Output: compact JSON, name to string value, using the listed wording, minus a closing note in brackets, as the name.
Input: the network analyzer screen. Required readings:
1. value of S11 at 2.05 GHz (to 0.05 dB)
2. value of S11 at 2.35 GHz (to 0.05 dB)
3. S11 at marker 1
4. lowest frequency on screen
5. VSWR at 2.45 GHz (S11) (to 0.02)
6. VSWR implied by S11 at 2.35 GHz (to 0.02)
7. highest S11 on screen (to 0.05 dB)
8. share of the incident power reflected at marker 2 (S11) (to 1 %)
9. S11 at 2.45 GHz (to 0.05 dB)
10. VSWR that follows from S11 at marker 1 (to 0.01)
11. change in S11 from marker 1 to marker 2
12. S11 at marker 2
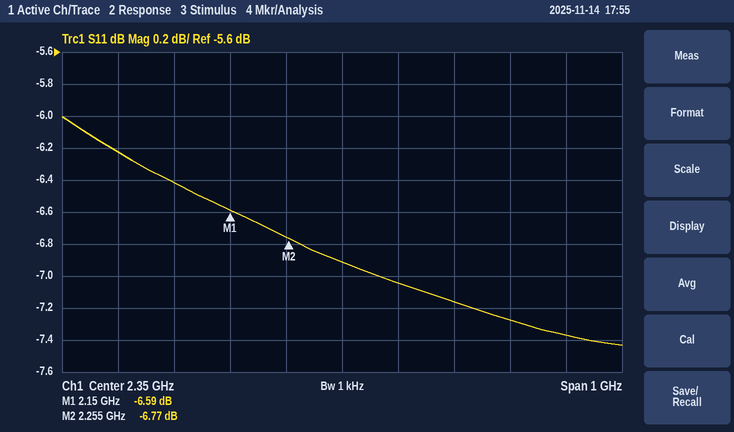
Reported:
{"value of S11 at 2.05 GHz": "-6.40 dB", "value of S11 at 2.35 GHz": "-6.90 dB", "S11 at marker 1": "-6.59 dB", "lowest frequency on screen": "1.85 GHz", "VSWR at 2.45 GHz (S11)": "2.60", "VSWR implied by S11 at 2.35 GHz": "2.64", "highest S11 on screen": "-6.00 dB", "share of the incident power reflected at marker 2 (S11)": "21 %", "S11 at 2.45 GHz": "-7.05 dB", "VSWR that follows from S11 at marker 1": "2.76", "change in S11 from marker 1 to marker 2": "-0.18 dB", "S11 at marker 2": "-6.77 dB"}
